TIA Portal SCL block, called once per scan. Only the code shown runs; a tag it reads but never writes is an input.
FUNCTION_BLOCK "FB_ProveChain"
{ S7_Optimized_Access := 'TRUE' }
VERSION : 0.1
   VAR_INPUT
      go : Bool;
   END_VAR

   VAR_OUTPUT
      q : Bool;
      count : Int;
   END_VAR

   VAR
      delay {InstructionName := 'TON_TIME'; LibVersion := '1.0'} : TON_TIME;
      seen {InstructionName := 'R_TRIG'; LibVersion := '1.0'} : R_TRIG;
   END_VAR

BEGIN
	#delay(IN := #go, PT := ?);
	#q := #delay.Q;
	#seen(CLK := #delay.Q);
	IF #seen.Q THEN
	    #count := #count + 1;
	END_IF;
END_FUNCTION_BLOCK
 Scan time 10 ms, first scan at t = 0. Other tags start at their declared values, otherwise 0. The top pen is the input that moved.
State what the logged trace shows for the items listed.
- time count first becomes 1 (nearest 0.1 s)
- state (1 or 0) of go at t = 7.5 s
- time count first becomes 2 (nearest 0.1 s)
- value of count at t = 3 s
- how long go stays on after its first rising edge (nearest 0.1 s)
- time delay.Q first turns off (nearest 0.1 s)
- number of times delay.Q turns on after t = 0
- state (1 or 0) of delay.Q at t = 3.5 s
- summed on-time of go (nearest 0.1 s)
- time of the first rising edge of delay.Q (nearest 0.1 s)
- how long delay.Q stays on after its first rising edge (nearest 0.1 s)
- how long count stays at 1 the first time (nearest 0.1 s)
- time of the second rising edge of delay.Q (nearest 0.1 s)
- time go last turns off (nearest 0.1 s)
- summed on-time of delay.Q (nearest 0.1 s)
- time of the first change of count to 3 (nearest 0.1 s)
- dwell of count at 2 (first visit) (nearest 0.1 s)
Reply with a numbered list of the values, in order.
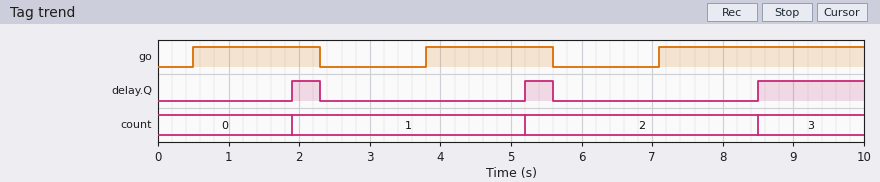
1. 1.9 s
2. 1
3. 5.2 s
4. 1
5. 1.8 s
6. 2.3 s
7. 3
8. 0
9. 6.5 s
10. 1.9 s
11. 0.4 s
12. 3.3 s
13. 5.2 s
14. 5.6 s
15. 2.3 s
16. 8.5 s
17. 3.3 s
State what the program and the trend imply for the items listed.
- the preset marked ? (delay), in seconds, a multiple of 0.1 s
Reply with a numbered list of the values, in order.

1. 1.4 s
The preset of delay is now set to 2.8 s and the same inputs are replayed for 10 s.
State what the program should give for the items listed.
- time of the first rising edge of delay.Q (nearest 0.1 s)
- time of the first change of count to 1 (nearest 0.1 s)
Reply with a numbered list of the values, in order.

1. 9.9 s
2. 9.9 s
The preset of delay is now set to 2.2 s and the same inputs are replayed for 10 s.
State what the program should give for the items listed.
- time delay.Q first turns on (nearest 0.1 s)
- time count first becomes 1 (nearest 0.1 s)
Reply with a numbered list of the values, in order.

1. 9.3 s
2. 9.3 s
